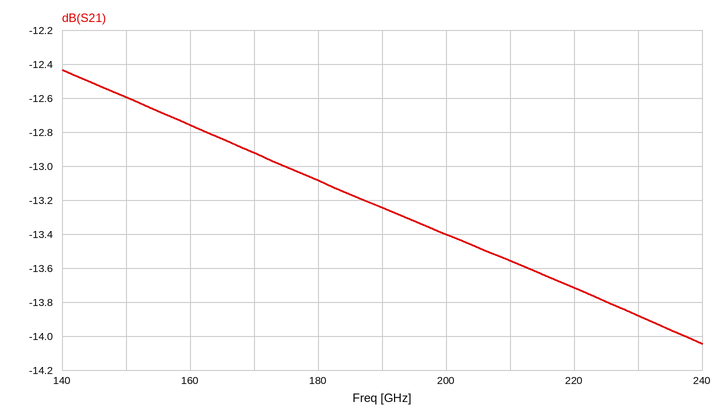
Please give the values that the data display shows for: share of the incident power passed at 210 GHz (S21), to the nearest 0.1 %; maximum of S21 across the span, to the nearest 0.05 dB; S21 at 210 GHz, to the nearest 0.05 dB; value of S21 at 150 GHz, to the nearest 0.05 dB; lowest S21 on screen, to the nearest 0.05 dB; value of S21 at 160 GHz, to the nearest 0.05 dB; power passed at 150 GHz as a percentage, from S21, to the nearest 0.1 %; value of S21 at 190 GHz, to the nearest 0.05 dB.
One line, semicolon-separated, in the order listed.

4.4 %; -12.45 dB; -13.55 dB; -12.60 dB; -14.05 dB; -12.75 dB; 5.5 %; -13.25 dB
